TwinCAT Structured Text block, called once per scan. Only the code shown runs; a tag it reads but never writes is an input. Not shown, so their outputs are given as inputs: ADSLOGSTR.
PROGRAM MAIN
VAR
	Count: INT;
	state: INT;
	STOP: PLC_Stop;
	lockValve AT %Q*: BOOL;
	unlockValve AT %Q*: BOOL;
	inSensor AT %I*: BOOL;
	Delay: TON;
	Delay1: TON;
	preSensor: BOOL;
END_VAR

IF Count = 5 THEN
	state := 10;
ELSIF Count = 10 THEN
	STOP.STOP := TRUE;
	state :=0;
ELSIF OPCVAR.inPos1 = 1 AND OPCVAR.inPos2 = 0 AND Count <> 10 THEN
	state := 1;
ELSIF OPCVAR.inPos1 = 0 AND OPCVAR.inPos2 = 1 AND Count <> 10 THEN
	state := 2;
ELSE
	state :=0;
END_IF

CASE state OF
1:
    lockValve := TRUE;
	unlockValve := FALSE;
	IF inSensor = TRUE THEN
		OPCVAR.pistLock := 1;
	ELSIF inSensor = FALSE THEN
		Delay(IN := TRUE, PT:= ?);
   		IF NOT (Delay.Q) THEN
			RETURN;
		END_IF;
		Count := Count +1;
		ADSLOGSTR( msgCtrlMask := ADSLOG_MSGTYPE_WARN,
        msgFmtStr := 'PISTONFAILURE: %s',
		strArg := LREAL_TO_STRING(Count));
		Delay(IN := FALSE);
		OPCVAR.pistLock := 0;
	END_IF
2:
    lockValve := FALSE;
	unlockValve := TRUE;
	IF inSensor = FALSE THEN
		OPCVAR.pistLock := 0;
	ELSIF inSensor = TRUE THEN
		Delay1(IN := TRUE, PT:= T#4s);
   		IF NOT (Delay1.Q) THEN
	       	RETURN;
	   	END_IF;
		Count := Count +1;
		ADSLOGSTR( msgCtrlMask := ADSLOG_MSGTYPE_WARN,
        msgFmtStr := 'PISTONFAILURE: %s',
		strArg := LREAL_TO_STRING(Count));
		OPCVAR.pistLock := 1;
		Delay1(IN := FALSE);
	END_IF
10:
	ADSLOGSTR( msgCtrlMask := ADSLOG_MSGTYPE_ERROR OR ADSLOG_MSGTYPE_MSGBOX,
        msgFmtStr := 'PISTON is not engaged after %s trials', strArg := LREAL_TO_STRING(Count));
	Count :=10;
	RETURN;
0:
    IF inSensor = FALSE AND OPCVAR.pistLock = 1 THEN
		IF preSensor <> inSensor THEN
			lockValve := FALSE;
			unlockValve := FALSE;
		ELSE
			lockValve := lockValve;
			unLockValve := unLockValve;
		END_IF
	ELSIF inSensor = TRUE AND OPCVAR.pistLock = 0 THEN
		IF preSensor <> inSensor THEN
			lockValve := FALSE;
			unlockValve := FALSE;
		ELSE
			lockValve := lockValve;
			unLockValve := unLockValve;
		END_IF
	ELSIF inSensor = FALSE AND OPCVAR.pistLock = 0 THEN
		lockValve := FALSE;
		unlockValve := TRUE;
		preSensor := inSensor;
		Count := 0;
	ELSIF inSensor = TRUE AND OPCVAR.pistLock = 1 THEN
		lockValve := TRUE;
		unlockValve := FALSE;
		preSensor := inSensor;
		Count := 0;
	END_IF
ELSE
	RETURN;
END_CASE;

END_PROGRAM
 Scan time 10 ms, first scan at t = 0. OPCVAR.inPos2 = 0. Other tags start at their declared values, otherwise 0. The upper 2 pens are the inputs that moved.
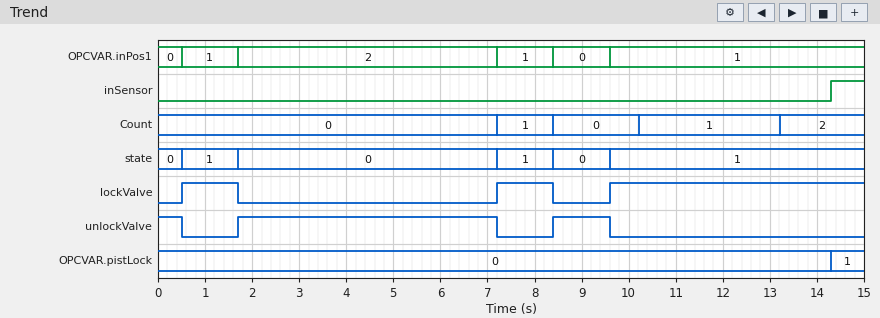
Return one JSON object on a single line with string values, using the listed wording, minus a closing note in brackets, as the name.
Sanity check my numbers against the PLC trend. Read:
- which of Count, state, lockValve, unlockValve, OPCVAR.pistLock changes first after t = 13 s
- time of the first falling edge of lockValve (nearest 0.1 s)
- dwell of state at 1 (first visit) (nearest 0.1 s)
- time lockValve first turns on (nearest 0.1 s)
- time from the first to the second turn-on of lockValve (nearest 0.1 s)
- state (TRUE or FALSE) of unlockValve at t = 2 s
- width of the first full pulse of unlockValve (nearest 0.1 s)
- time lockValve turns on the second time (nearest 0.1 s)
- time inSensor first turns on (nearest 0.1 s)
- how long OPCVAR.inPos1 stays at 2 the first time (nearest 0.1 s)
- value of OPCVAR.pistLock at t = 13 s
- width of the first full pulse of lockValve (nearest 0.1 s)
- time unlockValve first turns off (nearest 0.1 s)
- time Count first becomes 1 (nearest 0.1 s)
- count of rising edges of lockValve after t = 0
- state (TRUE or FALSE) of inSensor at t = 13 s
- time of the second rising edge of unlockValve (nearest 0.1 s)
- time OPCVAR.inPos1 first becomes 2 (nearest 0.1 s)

{"which of Count, state, lockValve, unlockValve, OPCVAR.pistLock changes first after t = 13 s": "Count", "time of the first falling edge of lockValve": "1.7 s", "dwell of state at 1 (first visit)": "1.2 s", "time lockValve first turns on": "0.5 s", "time from the first to the second turn-on of lockValve": "6.7 s", "state (TRUE or FALSE) of unlockValve at t = 2 s": "TRUE", "width of the first full pulse of unlockValve": "5.5 s", "time lockValve turns on the second time": "7.2 s", "time inSensor first turns on": "14.3 s", "how long OPCVAR.inPos1 stays at 2 the first time": "5.5 s", "value of OPCVAR.pistLock at t = 13 s": "0", "width of the first full pulse of lockValve": "1.2 s", "time unlockValve first turns off": "0.5 s", "time Count first becomes 1": "7.2 s", "count of rising edges of lockValve after t = 0": "3", "state (TRUE or FALSE) of inSensor at t = 13 s": "FALSE", "time of the second rising edge of unlockValve": "8.4 s", "time OPCVAR.inPos1 first becomes 2": "1.7 s"}
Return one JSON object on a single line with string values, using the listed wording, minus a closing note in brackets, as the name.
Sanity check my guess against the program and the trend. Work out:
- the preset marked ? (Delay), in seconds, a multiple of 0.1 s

{"the preset marked ? (Delay), in seconds, a multiple of 0.1 s": "3.0 s"}
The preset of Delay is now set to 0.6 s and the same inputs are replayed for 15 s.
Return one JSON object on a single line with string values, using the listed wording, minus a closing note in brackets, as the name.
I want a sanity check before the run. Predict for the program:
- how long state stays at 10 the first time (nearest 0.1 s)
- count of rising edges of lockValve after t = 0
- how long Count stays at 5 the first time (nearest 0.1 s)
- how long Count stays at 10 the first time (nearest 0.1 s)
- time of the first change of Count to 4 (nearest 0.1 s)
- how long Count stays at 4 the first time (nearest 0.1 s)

{"how long state stays at 10 the first time": "0.0 s", "count of rising edges of lockValve after t = 0": "4", "how long Count stays at 5 the first time": "0.0 s", "how long Count stays at 10 the first time": "0.0 s", "time of the first change of Count to 4": "11.4 s", "how long Count stays at 4 the first time": "0.6 s"}
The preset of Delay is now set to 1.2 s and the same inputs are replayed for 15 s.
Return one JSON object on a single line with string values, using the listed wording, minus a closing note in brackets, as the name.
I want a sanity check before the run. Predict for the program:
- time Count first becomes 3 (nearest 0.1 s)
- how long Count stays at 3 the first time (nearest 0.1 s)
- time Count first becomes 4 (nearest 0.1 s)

{"time Count first becomes 3": "12.0 s", "how long Count stays at 3 the first time": "1.2 s", "time Count first becomes 4": "13.2 s"}
